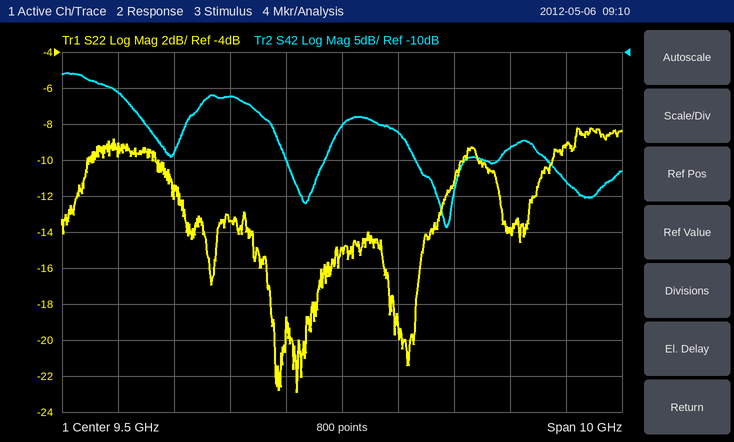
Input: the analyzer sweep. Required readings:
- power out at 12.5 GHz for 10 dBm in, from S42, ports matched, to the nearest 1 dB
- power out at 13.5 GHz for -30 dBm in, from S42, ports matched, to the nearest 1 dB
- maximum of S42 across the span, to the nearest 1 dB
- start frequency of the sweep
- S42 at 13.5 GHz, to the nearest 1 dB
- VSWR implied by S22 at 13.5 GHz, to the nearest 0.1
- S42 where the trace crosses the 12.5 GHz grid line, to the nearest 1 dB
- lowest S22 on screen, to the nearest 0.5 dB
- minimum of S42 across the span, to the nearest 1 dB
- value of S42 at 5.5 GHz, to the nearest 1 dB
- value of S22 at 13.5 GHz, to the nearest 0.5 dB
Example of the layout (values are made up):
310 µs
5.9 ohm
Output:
-13 dBm
-58 dBm
-13 dB
4.5 GHz
-28 dB
2.1
-23 dB
-23.0 dB
-34 dB
-16 dB
-9.0 dB
